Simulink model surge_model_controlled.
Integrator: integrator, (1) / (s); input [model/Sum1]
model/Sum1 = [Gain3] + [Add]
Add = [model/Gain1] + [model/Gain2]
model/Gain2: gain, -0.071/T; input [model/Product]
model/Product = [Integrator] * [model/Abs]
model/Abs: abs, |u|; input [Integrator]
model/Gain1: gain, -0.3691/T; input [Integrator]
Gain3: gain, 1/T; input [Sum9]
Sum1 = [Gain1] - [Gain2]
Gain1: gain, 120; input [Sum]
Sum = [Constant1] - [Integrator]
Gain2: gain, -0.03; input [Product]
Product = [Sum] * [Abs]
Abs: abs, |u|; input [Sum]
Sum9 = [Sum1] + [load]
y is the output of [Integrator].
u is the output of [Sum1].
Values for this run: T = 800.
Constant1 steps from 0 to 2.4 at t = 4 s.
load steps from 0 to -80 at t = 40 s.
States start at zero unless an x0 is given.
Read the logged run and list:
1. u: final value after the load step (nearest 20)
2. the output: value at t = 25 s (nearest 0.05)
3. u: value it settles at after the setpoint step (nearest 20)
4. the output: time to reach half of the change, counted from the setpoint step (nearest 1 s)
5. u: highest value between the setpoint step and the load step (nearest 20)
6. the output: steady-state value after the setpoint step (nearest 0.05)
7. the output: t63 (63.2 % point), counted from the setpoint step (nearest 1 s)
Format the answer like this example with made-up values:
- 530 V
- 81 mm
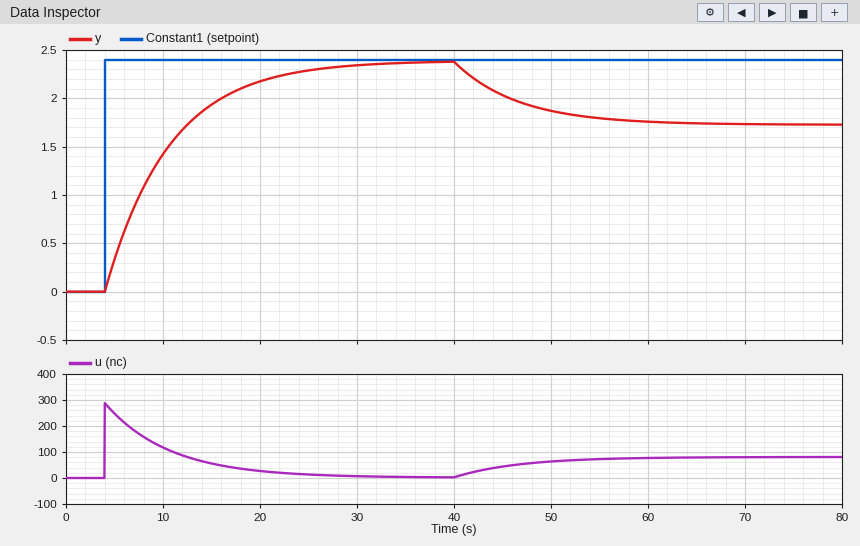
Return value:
- 80
- 2.30
- 0
- 5 s
- 280
- 2.40
- 7 s
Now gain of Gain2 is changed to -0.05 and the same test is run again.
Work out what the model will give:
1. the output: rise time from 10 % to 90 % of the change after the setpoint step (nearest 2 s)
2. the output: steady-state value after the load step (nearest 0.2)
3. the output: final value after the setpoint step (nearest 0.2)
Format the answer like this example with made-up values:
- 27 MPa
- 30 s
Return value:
- 14 s
- 1.8
- 2.4
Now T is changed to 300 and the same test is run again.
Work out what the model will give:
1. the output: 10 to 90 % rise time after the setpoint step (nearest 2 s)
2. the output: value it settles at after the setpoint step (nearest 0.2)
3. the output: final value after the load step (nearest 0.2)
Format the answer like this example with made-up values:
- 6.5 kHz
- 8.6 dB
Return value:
- 6 s
- 2.4
- 1.8
